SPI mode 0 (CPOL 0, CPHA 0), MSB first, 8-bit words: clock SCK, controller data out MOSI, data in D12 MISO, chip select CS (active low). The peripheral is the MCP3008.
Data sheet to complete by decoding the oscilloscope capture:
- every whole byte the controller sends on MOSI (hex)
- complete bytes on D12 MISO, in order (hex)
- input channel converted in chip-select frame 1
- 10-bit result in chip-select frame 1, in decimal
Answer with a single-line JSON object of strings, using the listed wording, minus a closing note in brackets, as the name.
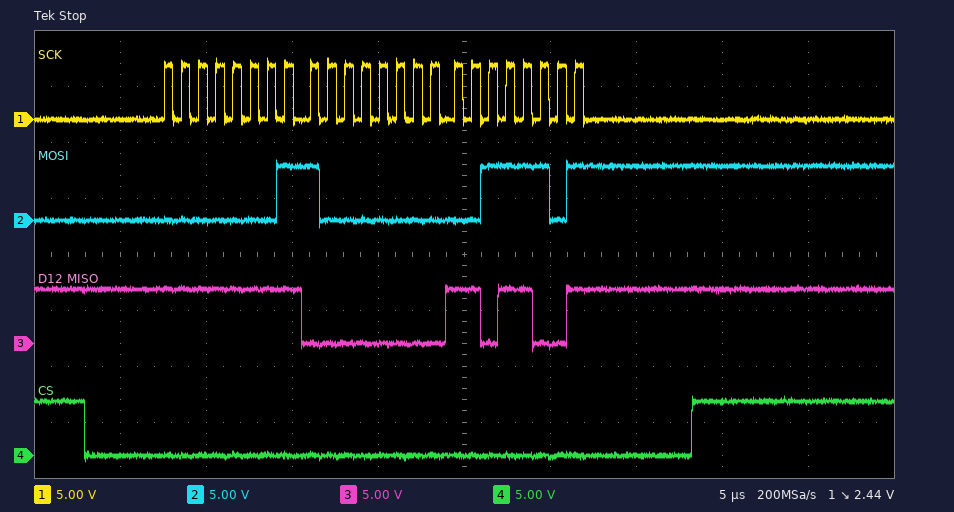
{"every whole byte the controller sends on MOSI": "01 80 3D", "complete bytes on D12 MISO, in order": "FF 00 D9", "input channel converted in chip-select frame 1": "0", "10-bit result in chip-select frame 1, in decimal": "217"}
